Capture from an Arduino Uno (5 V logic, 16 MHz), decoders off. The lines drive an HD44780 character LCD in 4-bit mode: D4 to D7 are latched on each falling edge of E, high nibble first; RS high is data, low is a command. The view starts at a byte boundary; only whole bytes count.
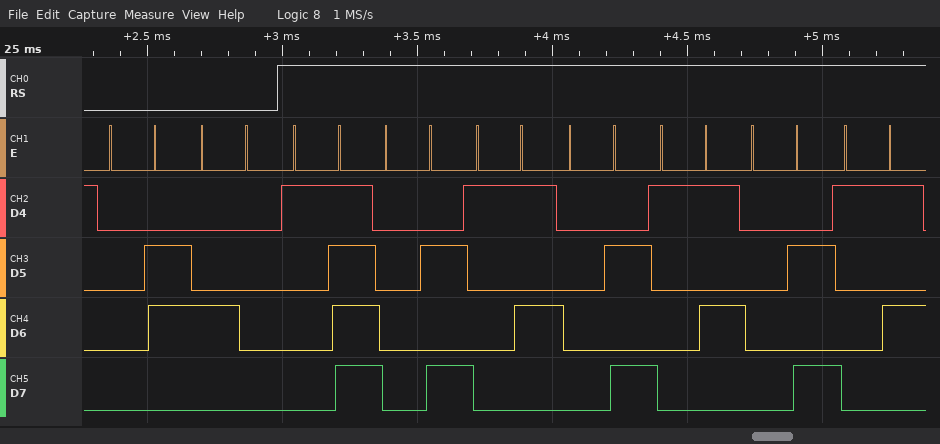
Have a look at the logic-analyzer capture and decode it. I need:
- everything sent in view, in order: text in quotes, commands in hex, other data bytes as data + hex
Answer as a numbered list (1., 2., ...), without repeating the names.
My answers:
1. 0x06 0x40 data 1F 0A 15 0A 15 0A 15
